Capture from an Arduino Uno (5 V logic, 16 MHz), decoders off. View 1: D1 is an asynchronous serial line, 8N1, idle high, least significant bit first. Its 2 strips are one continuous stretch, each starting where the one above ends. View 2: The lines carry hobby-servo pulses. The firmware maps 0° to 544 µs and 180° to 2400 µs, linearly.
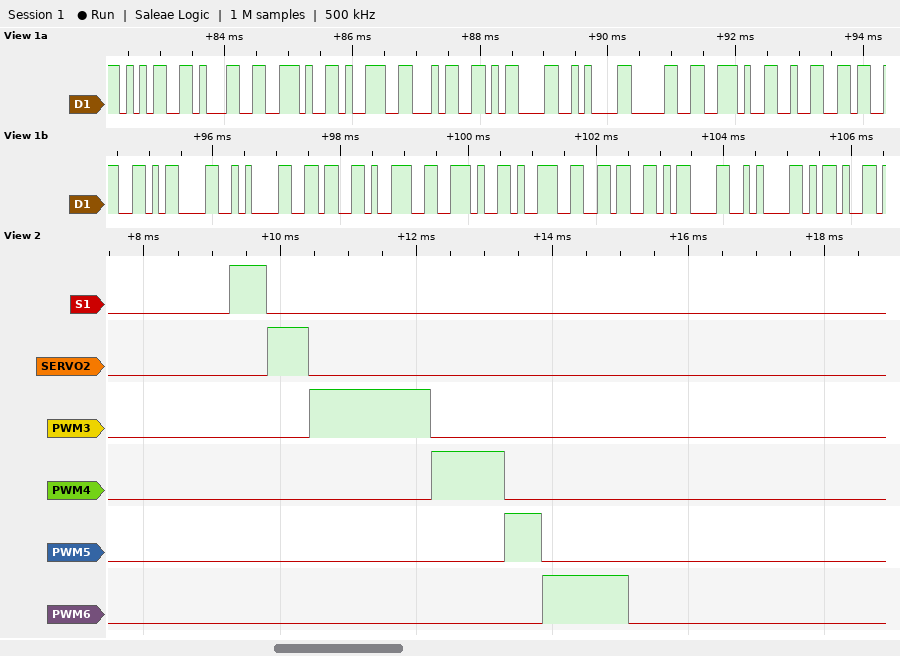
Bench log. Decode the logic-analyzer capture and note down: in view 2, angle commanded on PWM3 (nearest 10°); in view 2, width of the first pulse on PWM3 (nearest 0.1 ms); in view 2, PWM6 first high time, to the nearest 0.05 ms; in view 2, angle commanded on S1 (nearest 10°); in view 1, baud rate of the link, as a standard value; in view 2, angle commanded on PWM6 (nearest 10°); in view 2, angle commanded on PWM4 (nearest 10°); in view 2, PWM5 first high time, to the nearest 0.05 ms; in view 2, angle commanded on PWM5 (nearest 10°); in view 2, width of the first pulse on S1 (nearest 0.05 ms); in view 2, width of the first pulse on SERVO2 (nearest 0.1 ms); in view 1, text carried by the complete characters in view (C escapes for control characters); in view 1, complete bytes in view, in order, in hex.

120°
1.8 ms
1.25 ms
0°
9600 baud
70°
50°
0.55 ms
0°
0.55 ms
0.6 ms
"51.94\r\n0.23\r\n69.96\r\n-"
0x35 0x31 0x2E 0x39 0x34 0x0D 0x0A 0x30 0x2E 0x32 0x33 0x0D 0x0A 0x36 0x39 0x2E 0x39 0x36 0x0D 0x0A 0x2D
